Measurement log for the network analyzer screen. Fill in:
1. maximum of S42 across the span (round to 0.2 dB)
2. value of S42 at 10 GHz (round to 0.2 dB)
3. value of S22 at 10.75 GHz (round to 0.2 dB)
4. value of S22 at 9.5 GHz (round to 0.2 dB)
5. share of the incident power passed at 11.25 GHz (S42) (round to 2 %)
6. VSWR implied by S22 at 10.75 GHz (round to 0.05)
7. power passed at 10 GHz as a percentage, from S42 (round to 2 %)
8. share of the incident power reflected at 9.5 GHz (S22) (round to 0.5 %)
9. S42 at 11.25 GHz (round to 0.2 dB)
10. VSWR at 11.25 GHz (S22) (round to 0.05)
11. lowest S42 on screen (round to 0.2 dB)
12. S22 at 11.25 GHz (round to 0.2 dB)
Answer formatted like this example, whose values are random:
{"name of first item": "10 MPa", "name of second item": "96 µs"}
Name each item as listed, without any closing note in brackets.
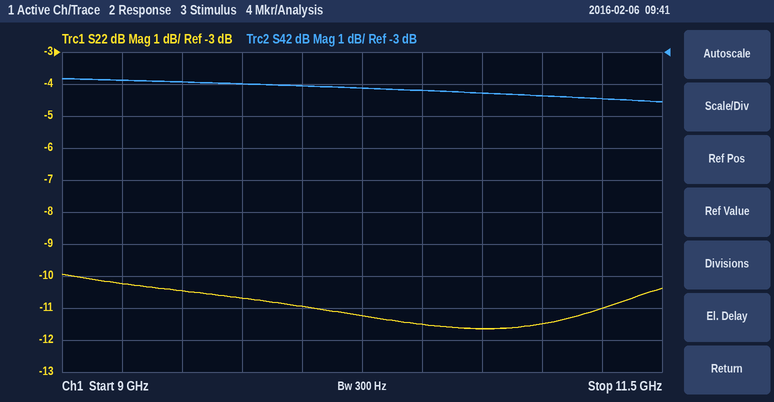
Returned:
{"maximum of S42 across the span": "-3.8 dB", "value of S42 at 10 GHz": "-4.0 dB", "value of S22 at 10.75 GHz": "-11.6 dB", "value of S22 at 9.5 GHz": "-10.4 dB", "share of the incident power passed at 11.25 GHz (S42)": "36 %", "VSWR implied by S22 at 10.75 GHz": "1.70", "power passed at 10 GHz as a percentage, from S42": "40 %", "share of the incident power reflected at 9.5 GHz (S22)": "9.0 %", "S42 at 11.25 GHz": "-4.4 dB", "VSWR at 11.25 GHz (S22)": "1.80", "lowest S42 on screen": "-4.6 dB", "S22 at 11.25 GHz": "-11.0 dB"}
